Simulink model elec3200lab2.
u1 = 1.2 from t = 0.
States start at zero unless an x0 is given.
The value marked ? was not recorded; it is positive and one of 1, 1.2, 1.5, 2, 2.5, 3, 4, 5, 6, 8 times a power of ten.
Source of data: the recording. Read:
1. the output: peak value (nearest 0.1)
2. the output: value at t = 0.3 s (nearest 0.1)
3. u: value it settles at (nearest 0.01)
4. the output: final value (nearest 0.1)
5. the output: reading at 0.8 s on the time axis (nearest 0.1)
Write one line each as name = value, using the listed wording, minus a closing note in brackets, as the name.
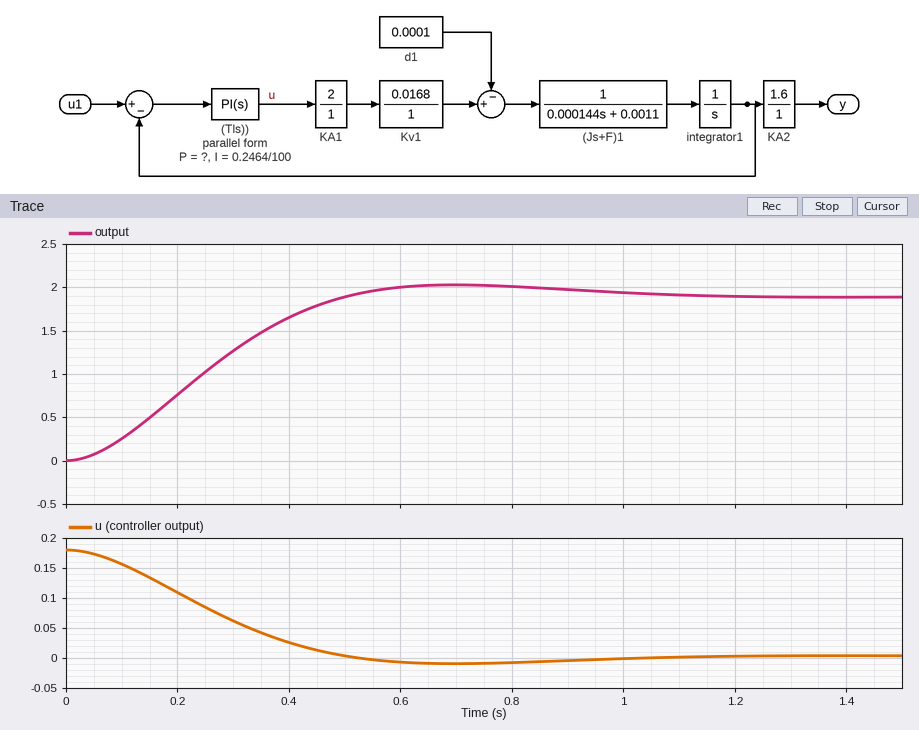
the output: peak value = 2.0
the output: value at t = 0.3 s = 1.3
u: value it settles at = 0.00
the output: final value = 1.9
the output: reading at 0.8 s on the time axis = 2.0
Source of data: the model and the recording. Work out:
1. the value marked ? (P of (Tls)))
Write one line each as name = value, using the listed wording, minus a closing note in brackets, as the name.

the value marked ? (P of (Tls))) = 0.15
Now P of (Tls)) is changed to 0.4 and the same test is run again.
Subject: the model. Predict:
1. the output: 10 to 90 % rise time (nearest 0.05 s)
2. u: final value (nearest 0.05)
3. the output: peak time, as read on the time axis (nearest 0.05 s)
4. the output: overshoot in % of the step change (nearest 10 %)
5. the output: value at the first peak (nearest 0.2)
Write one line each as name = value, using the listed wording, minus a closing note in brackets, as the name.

the output: 10 to 90 % rise time = 0.15 s
u: final value = 0.00
the output: peak time, as read on the time axis = 0.35 s
the output: overshoot in % of the step change = 30 %
the output: value at the first peak = 2.4
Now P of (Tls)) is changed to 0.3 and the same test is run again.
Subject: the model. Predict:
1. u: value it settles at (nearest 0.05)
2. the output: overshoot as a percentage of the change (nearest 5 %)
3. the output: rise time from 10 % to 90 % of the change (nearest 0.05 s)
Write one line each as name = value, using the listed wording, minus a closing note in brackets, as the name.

u: value it settles at = 0.00
the output: overshoot as a percentage of the change = 20 %
the output: rise time from 10 % to 90 % of the change = 0.20 s
